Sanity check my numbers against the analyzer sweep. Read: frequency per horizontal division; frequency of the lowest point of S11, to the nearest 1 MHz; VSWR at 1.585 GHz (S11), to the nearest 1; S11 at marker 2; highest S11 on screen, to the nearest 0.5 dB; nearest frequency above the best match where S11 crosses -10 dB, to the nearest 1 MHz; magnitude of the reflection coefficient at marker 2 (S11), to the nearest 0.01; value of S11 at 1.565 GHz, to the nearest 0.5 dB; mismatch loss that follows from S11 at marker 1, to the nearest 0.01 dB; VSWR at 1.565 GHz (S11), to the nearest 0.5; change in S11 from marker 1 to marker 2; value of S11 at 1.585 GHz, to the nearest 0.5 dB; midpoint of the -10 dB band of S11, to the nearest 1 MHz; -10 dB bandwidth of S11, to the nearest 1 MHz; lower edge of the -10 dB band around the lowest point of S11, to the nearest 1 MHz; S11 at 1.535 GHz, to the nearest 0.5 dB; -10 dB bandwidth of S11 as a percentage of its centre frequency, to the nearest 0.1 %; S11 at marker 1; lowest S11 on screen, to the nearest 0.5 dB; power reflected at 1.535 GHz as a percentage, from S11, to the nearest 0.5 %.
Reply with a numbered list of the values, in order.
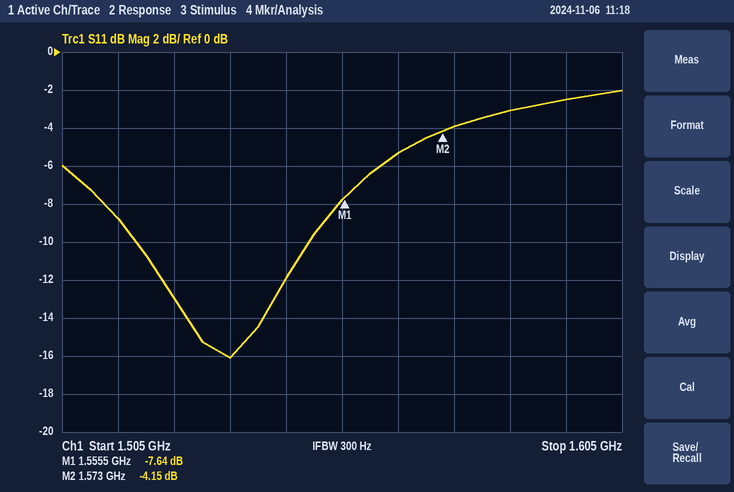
1. 10 MHz
2. 1.535 GHz
3. 6
4. -4.15 dB
5. -2.0 dB
6. 1.549 GHz
7. 0.62
8. -5.5 dB
9. 0.82 dB
10. 3.5
11. 3.49 dB
12. -3.0 dB
13. 1.534 GHz
14. 31 MHz
15. 1.518 GHz
16. -16.0 dB
17. 2.0 %
18. -7.64 dB
19. -16.0 dB
20. 2.5 %
